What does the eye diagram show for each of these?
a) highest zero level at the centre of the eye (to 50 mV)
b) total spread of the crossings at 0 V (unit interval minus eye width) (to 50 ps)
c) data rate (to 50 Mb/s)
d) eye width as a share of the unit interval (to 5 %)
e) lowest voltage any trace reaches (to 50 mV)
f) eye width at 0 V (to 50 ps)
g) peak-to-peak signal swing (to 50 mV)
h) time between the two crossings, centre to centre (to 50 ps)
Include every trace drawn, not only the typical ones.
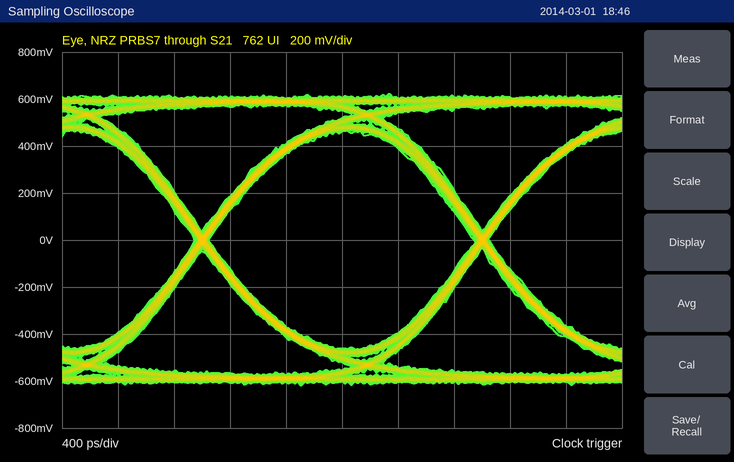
-450 mV
100 ps
500 Mb/s
95 %
-600 mV
1.90 ns
1.25 V
2.00 ns
